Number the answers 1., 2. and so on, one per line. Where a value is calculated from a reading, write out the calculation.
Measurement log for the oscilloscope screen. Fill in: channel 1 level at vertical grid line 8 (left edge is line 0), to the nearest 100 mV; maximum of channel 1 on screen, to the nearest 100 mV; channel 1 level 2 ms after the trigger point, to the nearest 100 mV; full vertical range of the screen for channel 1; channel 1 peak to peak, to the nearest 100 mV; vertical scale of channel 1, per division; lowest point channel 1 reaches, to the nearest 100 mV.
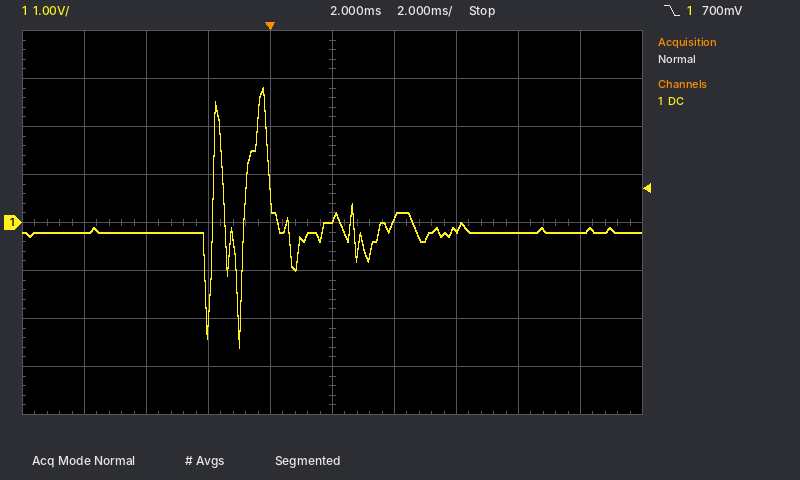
1. -200 mV
2. 2.8 V
3. 100 mV
4. 8 V
5. 2.8 V − (-2.6 V) = 5.4 V
6. 1 V
7. -2.6 V
